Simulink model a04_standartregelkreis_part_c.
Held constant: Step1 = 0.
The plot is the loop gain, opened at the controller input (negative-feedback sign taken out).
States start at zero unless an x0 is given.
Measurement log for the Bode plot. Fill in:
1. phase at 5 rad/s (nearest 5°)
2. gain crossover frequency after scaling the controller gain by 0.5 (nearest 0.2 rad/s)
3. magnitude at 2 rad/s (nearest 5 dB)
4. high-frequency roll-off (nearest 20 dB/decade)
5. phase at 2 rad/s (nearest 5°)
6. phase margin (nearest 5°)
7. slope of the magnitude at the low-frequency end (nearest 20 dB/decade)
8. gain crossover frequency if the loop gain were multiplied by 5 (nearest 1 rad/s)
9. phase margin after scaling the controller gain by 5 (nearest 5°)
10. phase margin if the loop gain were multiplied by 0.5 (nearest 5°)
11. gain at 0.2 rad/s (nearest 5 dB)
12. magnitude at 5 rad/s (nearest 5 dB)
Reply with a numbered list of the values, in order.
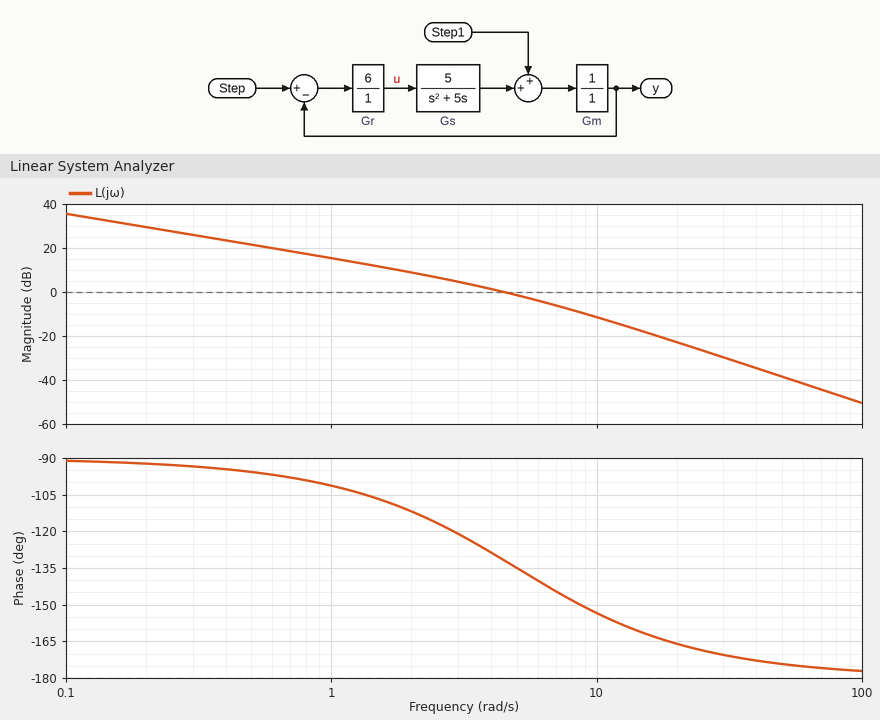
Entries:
1. -135°
2. 2.6 rad/s
3. 10 dB
4. -40 dB/decade
5. -110°
6. 50°
7. -20 dB/decade
8. 12 rad/s
9. 25°
10. 60°
11. 30 dB
12. 0 dB
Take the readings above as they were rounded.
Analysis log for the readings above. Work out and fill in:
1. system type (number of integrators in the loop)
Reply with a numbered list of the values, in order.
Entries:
1. 1
